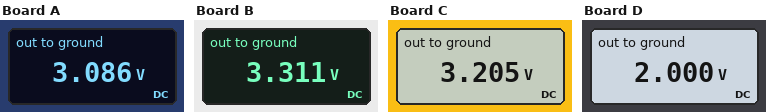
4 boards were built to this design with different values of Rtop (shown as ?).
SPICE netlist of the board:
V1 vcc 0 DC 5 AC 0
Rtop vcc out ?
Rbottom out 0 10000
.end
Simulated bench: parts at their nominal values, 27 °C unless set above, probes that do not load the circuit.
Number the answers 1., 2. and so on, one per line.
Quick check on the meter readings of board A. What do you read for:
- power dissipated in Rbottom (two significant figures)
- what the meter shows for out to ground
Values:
1. 950 µW
2. 3.086 V
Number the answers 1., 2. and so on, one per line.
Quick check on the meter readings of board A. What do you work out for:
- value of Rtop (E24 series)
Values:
1. 6.2 kΩ
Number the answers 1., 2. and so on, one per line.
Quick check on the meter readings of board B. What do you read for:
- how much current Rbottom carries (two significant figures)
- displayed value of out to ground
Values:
1. 330 µA
2. 3.311 V
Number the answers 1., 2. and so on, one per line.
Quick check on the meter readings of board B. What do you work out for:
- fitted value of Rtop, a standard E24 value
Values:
1. 5.1 kΩ
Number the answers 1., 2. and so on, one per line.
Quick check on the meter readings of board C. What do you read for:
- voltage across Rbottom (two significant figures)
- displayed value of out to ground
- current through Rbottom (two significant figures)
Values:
1. 3.2 V
2. 3.205 V
3. 320 µA
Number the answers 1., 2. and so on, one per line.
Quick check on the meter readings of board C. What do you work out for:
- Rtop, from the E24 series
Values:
1. 5.6 kΩ
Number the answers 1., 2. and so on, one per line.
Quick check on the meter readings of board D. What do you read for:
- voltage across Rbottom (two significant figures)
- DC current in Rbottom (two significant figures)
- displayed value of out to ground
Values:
1. 2.0 V
2. 200 µA
3. 2.000 V
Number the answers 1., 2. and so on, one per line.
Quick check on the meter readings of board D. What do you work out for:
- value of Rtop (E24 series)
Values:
1. 15 kΩ
